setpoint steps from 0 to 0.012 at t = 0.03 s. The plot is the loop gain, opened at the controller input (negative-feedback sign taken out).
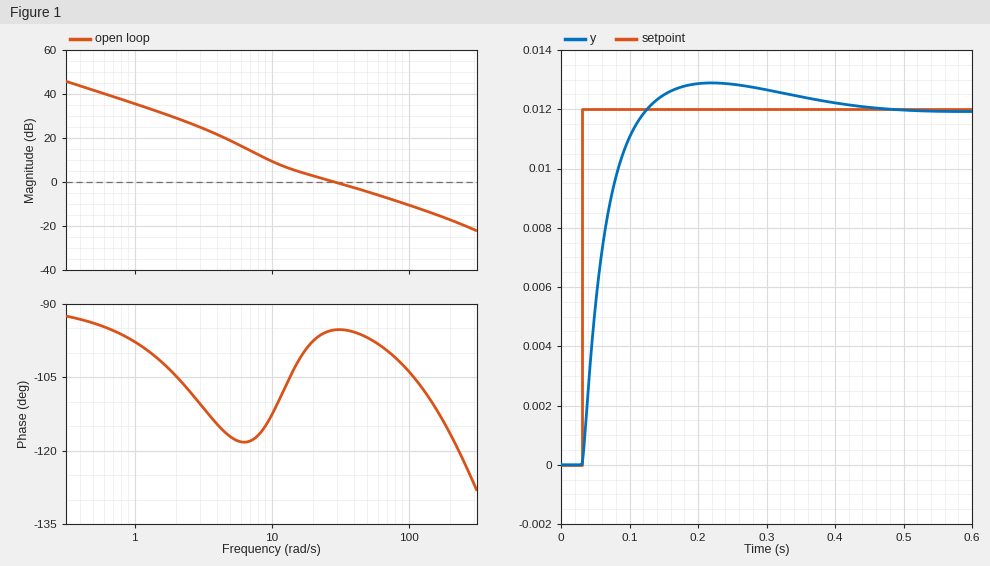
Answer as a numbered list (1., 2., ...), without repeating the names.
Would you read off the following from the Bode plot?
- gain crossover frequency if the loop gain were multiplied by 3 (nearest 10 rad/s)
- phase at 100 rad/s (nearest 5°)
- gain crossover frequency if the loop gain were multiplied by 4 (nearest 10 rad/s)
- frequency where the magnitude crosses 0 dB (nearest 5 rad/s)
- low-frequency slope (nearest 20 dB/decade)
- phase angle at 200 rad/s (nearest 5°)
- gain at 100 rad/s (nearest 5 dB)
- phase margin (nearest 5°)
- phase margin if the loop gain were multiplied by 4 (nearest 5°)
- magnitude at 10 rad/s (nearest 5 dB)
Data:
1. 90 rad/s
2. -105°
3. 120 rad/s
4. 30 rad/s
5. -20 dB/decade
6. -115°
7. -10 dB
8. 85°
9. 75°
10. 10 dB
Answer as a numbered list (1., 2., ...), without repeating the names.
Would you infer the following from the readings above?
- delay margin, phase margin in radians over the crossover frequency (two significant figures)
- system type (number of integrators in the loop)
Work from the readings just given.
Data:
1. 0.049 s
2. 1
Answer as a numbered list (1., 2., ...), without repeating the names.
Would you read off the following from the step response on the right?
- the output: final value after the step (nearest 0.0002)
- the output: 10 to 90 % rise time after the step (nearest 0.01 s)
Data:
1. 0.0120
2. 0.06 s
